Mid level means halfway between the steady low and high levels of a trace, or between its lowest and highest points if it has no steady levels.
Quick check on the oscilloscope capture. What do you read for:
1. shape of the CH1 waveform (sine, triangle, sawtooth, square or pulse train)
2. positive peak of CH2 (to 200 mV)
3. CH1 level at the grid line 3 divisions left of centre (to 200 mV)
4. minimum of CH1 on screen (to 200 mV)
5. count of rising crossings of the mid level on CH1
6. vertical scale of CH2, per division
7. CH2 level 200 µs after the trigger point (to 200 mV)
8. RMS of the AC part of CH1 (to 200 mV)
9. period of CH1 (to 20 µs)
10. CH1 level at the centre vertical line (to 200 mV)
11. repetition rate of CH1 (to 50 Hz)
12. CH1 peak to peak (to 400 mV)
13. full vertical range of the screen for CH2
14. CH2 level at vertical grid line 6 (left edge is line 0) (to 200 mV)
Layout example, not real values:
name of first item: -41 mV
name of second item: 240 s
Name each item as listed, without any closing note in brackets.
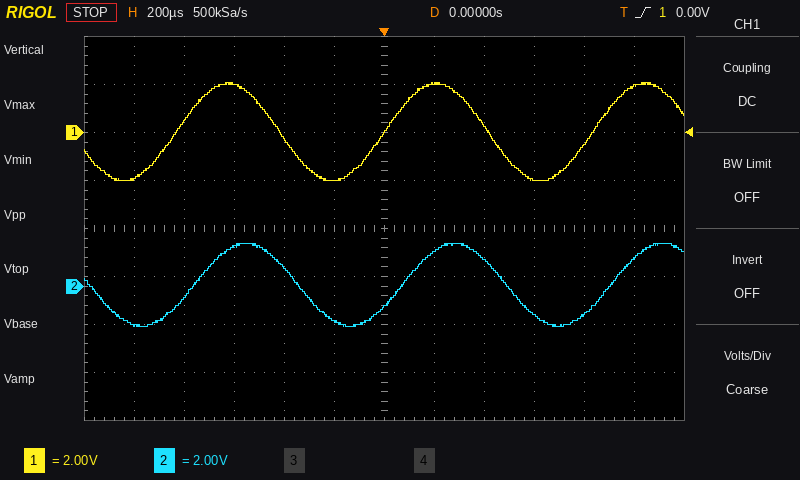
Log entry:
shape of the CH1 waveform: sine
positive peak of CH2: 1.8 V
CH1 level at the grid line 3 divisions left of centre: 2.0 V
minimum of CH1 on screen: -2.0 V
count of rising crossings of the mid level on CH1: 3
vertical scale of CH2, per division: 2 V
CH2 level 200 µs after the trigger point: 1.4 V
RMS of the AC part of CH1: 1.4 V
period of CH1: 840 µs
CH1 level at the centre vertical line: 0.0 V
repetition rate of CH1: 1.20 kHz
CH1 peak to peak: 4.0 V
full vertical range of the screen for CH2: 16 V
CH2 level at vertical grid line 6 (left edge is line 0): -800 mV
